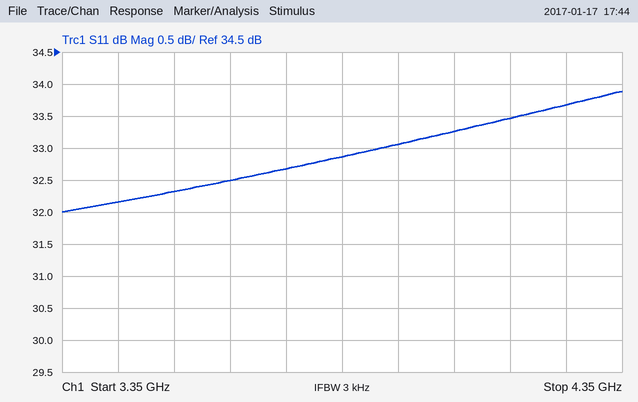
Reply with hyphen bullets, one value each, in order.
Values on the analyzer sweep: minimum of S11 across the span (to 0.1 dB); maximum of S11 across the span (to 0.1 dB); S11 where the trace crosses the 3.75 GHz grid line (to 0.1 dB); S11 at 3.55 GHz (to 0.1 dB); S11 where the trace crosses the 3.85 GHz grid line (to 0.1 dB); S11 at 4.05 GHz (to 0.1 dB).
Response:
- 32.0 dB
- 33.9 dB
- 32.7 dB
- 32.3 dB
- 32.9 dB
- 33.3 dB
